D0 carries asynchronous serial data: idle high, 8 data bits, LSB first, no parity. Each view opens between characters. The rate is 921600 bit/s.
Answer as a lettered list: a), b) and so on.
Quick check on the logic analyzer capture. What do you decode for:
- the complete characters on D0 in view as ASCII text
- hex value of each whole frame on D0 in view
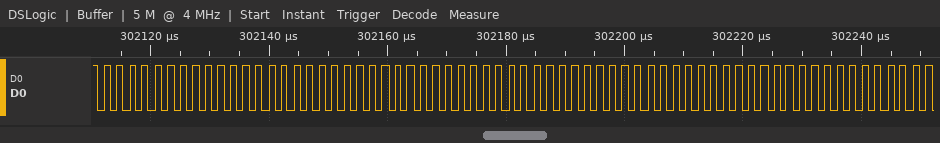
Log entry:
a) "UUUUUUUUUUUUU"
b) 55, 55, 55, 55, 55, 55, 55, 55, 55, 55, 55, 55, 55
